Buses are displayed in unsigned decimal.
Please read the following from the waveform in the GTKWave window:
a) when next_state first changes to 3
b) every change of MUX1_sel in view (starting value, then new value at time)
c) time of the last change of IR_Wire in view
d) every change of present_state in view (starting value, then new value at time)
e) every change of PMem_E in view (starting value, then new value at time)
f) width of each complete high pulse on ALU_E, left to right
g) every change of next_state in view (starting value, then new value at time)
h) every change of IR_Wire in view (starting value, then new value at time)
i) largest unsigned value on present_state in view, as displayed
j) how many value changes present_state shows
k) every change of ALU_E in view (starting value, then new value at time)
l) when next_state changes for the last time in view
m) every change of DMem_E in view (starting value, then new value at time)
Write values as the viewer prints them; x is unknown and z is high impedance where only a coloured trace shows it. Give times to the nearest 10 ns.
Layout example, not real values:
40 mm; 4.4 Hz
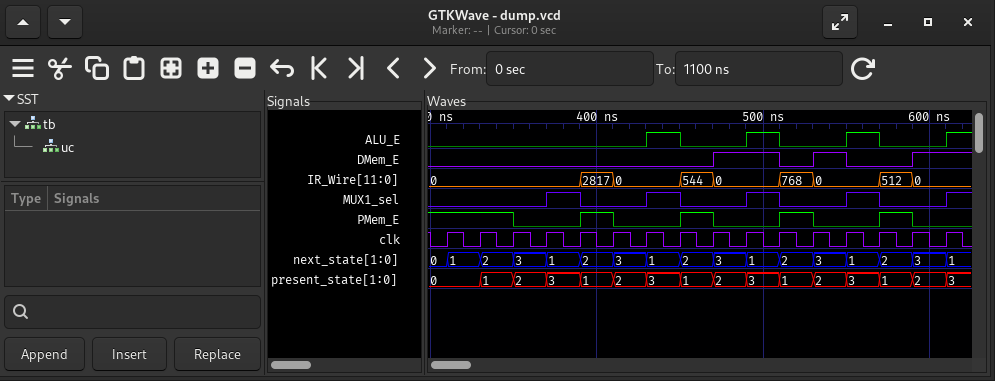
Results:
350 ns; 0, 1 at 370 ns, 0 at 390 ns, 1 at 430 ns, 0 at 450 ns, 1 at 490 ns, 0 at 510 ns, 1 at 550 ns, 0 at 570 ns, 1 at 610 ns; 590 ns; 0, 1 at 330 ns, 2 at 350 ns, 3 at 370 ns, 1 at 390 ns, 2 at 410 ns, 3 at 430 ns, 1 at 450 ns, 2 at 470 ns, 3 at 490 ns, 1 at 510 ns, 2 at 530 ns, 3 at 550 ns, 1 at 570 ns, 2 at 590 ns, 3 at 610 ns; 1, 0 at 350 ns, 1 at 390 ns, 0 at 410 ns, 1 at 450 ns, 0 at 470 ns, 1 at 510 ns, 0 at 530 ns, 1 at 570 ns, 0 at 590 ns; 20 ns, 20 ns, 20 ns; 0, 1 at 310 ns, 2 at 330 ns, 3 at 350 ns, 1 at 370 ns, 2 at 390 ns, 3 at 410 ns, 1 at 430 ns, 2 at 450 ns, 3 at 470 ns, 1 at 490 ns, 2 at 510 ns, 3 at 530 ns, 1 at 550 ns, 2 at 570 ns, 3 at 590 ns, 1 at 610 ns; 0, 2817 at 390 ns, 0 at 410 ns, 544 at 450 ns, 0 at 470 ns, 768 at 510 ns, 0 at 530 ns, 512 at 570 ns, 0 at 590 ns; 3; 15; 0, 1 at 430 ns, 0 at 450 ns, 1 at 490 ns, 0 at 510 ns, 1 at 550 ns, 0 at 570 ns, 1 at 610 ns; 610 ns; 0, 1 at 470 ns, 0 at 510 ns, 1 at 530 ns, 0 at 550 ns, 1 at 590 ns
